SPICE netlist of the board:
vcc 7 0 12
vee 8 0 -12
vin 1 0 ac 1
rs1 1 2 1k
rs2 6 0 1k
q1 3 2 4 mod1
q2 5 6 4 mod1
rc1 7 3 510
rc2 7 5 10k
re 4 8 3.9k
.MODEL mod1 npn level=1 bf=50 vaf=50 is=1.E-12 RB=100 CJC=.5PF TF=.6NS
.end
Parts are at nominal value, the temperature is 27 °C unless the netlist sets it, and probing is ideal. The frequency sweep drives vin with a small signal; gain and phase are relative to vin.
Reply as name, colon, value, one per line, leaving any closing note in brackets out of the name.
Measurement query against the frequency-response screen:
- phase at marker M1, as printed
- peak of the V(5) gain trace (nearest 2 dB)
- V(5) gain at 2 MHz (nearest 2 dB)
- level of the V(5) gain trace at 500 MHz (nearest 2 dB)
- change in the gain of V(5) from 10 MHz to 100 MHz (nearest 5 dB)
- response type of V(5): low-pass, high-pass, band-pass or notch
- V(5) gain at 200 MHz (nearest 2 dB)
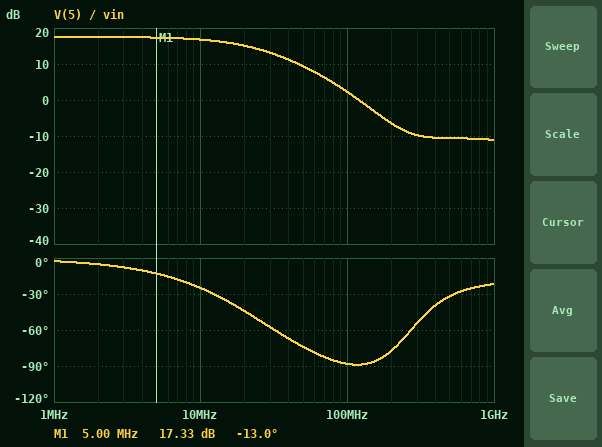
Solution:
phase at marker M1, as printed: -13.0 deg
peak of the V(5) gain trace: 18 dB
V(5) gain at 2 MHz: 18 dB
level of the V(5) gain trace at 500 MHz: -10 dB
change in the gain of V(5) from 10 MHz to 100 MHz: -15 dB
response type of V(5): low-pass, high-pass, band-pass or notch: low-pass
V(5) gain at 200 MHz: -6 dB
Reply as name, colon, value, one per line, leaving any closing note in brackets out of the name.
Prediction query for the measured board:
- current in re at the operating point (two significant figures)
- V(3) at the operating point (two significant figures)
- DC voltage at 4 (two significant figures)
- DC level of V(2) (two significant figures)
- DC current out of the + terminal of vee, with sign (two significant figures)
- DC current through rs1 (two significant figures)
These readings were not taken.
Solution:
current in re at the operating point: 2.9 mA
V(3) at the operating point: 11 V
DC voltage at 4: -570 mV
DC level of V(2): -27 mV
DC current out of the + terminal of vee, with sign: -2.9 mA
DC current through rs1: 27 µA
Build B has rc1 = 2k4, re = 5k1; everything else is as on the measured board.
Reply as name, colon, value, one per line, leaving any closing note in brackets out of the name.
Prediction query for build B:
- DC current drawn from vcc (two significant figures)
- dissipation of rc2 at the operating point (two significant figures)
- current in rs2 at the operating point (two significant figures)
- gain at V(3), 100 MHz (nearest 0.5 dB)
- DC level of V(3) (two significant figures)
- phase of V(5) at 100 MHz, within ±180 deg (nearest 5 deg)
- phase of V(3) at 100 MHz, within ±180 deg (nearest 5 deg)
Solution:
DC current drawn from vcc: 2.2 mA
dissipation of rc2 at the operating point: 11 mW
current in rs2 at the operating point: 20 µA
gain at V(3), 100 MHz: 3.5 dB
DC level of V(3): 9.2 V
phase of V(5) at 100 MHz, within ±180 deg: -115 deg
phase of V(3) at 100 MHz, within ±180 deg: 100 deg
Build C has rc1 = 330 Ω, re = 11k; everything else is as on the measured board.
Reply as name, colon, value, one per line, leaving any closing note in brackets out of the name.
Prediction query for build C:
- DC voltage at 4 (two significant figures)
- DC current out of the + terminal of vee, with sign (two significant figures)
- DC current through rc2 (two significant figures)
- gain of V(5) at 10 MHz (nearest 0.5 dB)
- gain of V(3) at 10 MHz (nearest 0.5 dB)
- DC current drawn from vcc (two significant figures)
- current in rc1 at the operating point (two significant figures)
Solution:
DC voltage at 4: -520 mV
DC current out of the + terminal of vee, with sign: -1.0 mA
DC current through rc2: 490 µA
gain of V(5) at 10 MHz: 30.5 dB
gain of V(3) at 10 MHz: 1.0 dB
DC current drawn from vcc: 1.0 mA
current in rc1 at the operating point: 530 µA
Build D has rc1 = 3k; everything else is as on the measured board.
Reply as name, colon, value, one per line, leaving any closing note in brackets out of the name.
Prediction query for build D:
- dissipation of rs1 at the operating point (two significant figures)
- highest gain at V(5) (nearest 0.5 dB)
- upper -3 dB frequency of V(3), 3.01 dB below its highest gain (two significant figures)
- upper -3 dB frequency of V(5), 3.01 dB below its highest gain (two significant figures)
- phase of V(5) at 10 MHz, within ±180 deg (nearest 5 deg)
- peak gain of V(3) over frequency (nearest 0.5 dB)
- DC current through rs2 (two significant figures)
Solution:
dissipation of rs1 at the operating point: 810 nW
highest gain at V(5): 12.5 dB
upper -3 dB frequency of V(3), 3.01 dB below its highest gain: 40 MHz
upper -3 dB frequency of V(5), 3.01 dB below its highest gain: 30 MHz
phase of V(5) at 10 MHz, within ±180 deg: -20 deg
peak gain of V(3) over frequency: 13.0 dB
DC current through rs2: 31 µA
